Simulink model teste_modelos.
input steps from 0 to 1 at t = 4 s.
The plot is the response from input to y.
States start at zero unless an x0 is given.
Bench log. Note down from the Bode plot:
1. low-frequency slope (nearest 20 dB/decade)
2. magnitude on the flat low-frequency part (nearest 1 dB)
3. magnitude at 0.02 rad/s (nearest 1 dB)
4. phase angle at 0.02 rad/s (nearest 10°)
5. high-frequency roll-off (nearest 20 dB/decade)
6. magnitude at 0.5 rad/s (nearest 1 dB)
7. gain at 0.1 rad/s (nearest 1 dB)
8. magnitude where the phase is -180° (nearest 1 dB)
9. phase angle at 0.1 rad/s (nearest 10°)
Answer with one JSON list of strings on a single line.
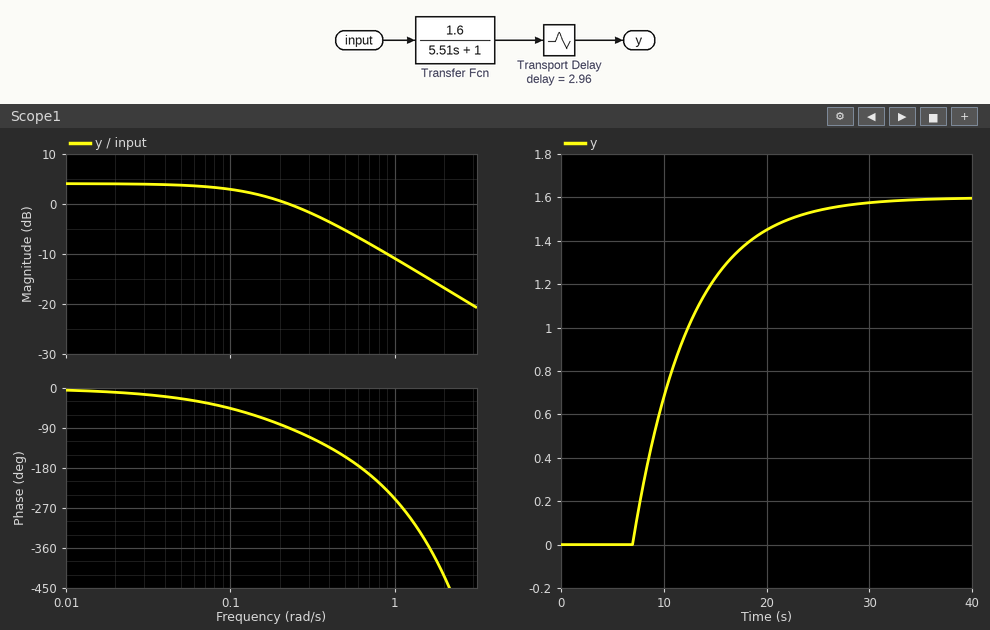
["0 dB/decade", "4 dB", "4 dB", "-10°", "-20 dB/decade", "-5 dB", "3 dB", "-7 dB", "-50°"]
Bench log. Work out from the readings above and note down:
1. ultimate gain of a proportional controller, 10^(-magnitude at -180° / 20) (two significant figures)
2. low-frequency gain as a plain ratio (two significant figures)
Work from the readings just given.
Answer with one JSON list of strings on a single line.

["2.2", "1.6"]
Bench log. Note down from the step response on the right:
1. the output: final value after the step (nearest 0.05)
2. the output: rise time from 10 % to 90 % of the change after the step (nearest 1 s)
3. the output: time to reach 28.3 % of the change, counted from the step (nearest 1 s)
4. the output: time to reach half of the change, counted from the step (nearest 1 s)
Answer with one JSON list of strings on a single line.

["1.60", "12 s", "5 s", "7 s"]
